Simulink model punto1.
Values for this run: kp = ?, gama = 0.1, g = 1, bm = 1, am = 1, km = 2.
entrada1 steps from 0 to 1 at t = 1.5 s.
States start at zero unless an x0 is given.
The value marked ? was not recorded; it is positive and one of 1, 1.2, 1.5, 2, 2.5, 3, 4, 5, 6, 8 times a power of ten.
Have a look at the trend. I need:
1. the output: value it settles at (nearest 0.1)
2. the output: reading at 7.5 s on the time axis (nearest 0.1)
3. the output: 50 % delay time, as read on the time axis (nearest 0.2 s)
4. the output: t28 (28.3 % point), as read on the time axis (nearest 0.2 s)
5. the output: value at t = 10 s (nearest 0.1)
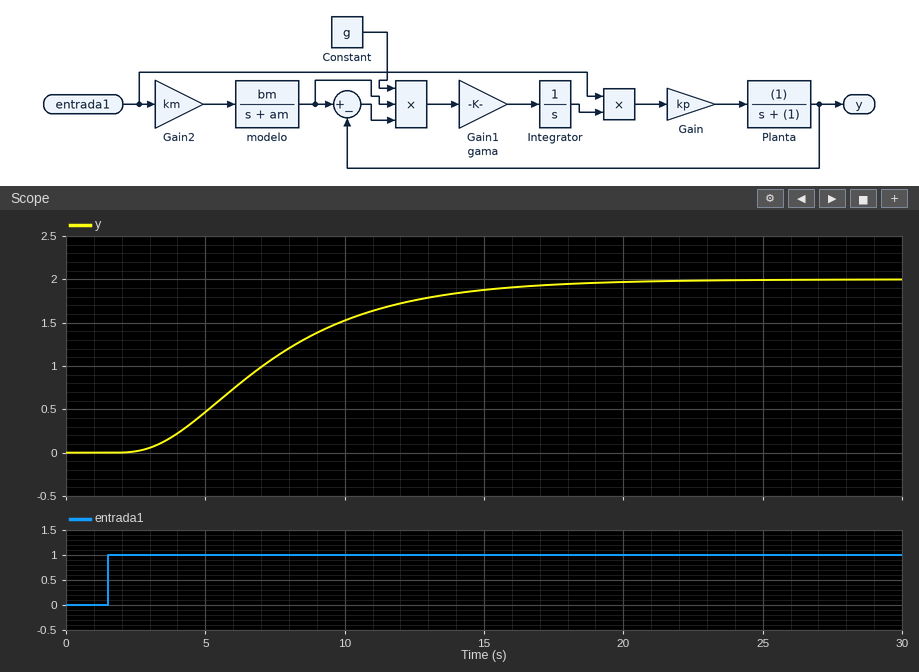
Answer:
2.0
1.1
7.0 s
5.4 s
1.5
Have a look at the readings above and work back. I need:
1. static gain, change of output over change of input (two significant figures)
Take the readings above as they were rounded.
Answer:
2.0
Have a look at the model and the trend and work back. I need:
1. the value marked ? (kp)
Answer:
1
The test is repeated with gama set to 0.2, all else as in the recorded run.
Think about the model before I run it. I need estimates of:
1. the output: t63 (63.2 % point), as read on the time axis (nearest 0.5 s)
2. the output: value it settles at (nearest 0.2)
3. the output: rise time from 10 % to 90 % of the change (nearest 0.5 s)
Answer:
6.0 s
2.0
4.5 s
